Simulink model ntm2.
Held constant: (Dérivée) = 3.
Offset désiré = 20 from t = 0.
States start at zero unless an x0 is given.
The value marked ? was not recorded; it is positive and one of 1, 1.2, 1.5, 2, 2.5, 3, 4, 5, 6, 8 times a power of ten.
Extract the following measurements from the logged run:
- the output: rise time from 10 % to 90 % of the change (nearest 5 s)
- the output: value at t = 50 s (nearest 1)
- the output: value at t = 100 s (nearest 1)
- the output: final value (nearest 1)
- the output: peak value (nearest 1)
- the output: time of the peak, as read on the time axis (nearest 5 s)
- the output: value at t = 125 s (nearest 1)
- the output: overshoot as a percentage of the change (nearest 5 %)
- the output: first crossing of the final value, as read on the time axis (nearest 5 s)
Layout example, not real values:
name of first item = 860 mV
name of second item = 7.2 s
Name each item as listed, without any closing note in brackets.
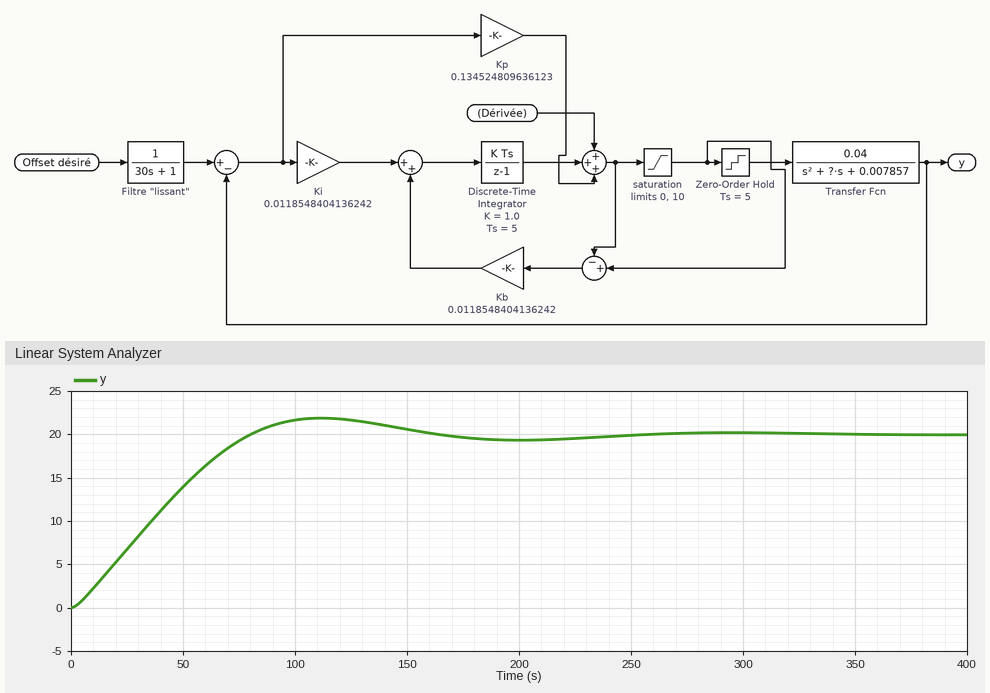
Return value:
the output: rise time from 10 % to 90 % of the change = 60 s
the output: value at t = 50 s = 14
the output: value at t = 100 s = 22
the output: final value = 20
the output: peak value = 22
the output: time of the peak, as read on the time axis = 110 s
the output: value at t = 125 s = 22
the output: overshoot as a percentage of the change = 10 %
the output: first crossing of the final value, as read on the time axis = 80 s
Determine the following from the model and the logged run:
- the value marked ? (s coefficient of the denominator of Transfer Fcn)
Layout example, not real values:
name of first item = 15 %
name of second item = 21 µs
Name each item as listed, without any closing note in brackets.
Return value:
the value marked ? = 0.4
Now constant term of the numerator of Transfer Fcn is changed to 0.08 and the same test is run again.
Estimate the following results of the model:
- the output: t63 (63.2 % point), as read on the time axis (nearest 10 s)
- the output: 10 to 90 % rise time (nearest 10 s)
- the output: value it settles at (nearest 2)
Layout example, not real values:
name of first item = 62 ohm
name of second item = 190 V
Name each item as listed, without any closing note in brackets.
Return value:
the output: t63 (63.2 % point), as read on the time axis = 30 s
the output: 10 to 90 % rise time = 40 s
the output: value it settles at = 20
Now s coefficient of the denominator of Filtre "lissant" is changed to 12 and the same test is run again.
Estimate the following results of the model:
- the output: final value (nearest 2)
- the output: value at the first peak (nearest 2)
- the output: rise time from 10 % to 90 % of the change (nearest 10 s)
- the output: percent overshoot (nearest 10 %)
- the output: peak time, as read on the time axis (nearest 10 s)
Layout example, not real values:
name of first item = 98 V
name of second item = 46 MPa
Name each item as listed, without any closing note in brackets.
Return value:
the output: final value = 20
the output: value at the first peak = 26
the output: rise time from 10 % to 90 % of the change = 40 s
the output: percent overshoot = 30 %
the output: peak time, as read on the time axis = 90 s
